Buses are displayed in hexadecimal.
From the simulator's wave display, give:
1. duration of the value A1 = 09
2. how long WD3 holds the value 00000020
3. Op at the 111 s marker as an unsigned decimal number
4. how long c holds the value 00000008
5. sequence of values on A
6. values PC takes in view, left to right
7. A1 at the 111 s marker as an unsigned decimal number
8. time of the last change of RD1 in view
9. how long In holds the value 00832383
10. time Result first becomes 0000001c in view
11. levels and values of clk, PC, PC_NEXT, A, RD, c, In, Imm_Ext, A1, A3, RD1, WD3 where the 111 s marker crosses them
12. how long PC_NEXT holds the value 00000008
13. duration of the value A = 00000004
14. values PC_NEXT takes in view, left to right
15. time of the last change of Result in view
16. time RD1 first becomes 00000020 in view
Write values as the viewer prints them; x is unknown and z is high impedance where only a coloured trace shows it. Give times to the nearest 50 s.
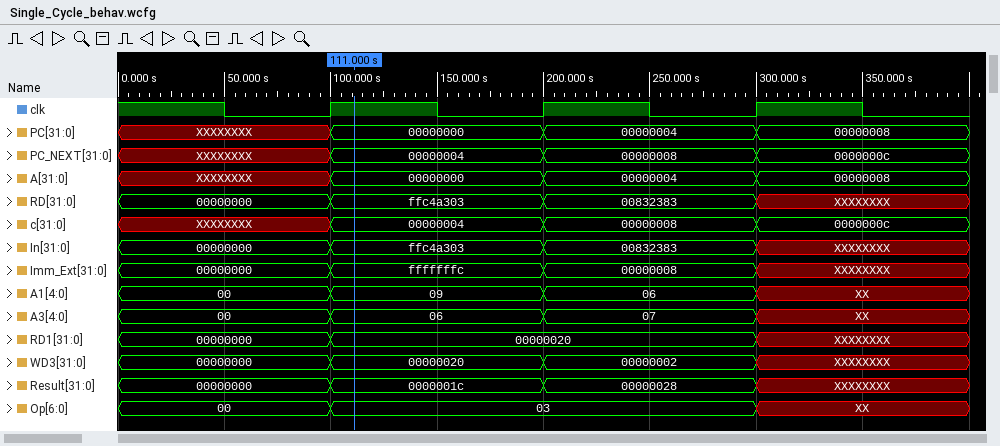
100 s
100 s
3
100 s
XXXXXXXX, 00000000, 00000004, 00000008
XXXXXXXX, 00000000, 00000004, 00000008
9
300 s
100 s
100 s
clk=1, PC=00000000, PC_NEXT=00000004, A=00000000, RD=ffc4a303, c=00000004, In=ffc4a303, Imm_Ext=fffffffc, A1=09, A3=06, RD1=00000020, WD3=00000020
100 s
100 s
XXXXXXXX, 00000004, 00000008, 0000000c
300 s
100 s
